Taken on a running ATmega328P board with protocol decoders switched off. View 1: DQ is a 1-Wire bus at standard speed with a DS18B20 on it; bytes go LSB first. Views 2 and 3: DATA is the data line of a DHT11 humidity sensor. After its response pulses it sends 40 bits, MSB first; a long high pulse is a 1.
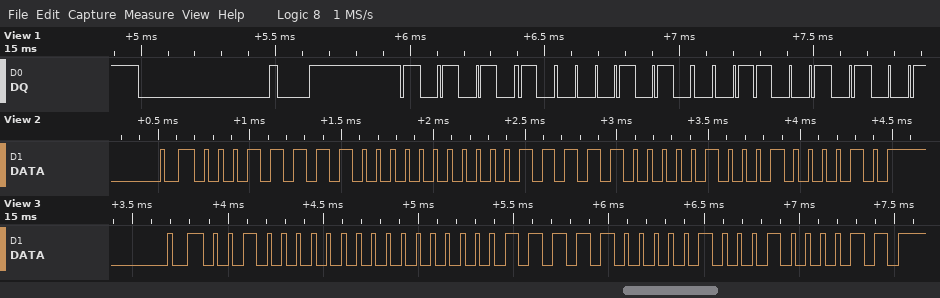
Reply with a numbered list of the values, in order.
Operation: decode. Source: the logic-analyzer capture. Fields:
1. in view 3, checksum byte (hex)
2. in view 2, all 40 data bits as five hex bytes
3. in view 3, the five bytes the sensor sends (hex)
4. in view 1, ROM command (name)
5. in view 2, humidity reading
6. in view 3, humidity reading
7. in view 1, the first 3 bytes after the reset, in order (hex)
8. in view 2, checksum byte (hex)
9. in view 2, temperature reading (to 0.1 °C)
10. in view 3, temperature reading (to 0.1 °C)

1. 0x43
2. 1F 00 1F 04 42
3. 20 00 1F 04 43
4. Match ROM
5. 31 %
6. 32 %
7. 55 28 A6
8. 0x42
9. 31.4 °C
10. 31.4 °C
